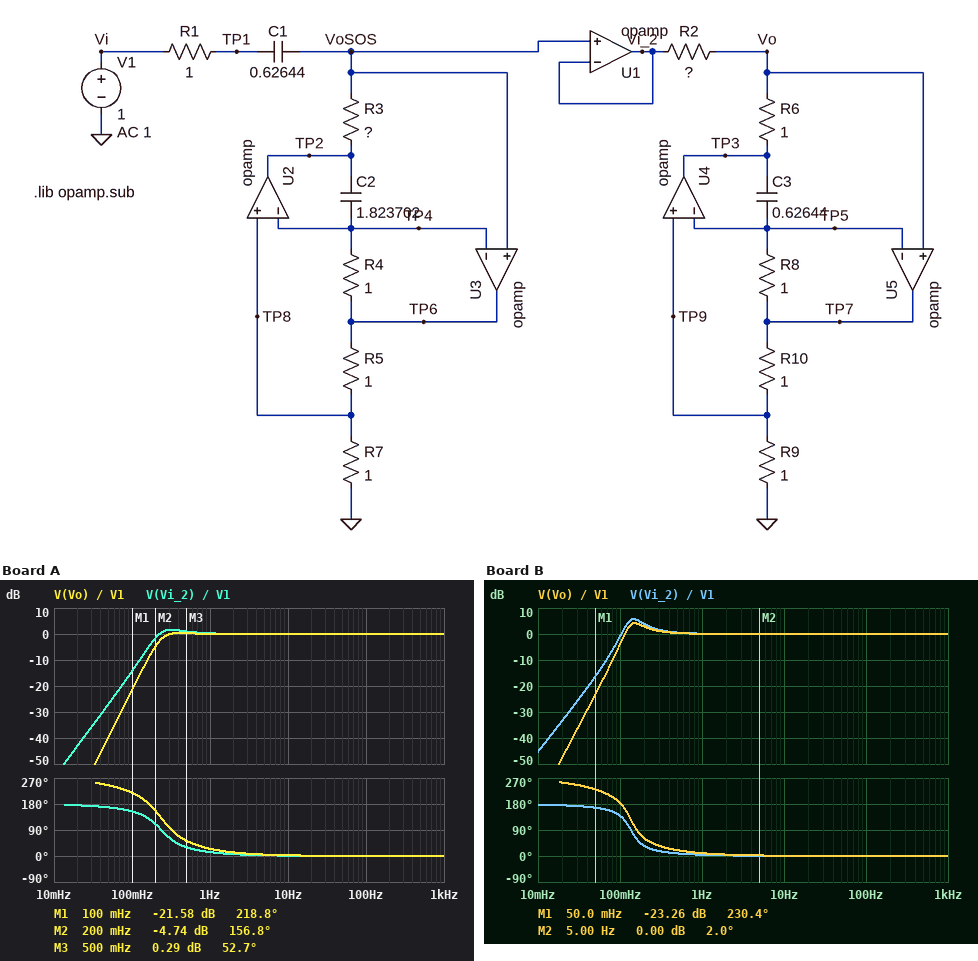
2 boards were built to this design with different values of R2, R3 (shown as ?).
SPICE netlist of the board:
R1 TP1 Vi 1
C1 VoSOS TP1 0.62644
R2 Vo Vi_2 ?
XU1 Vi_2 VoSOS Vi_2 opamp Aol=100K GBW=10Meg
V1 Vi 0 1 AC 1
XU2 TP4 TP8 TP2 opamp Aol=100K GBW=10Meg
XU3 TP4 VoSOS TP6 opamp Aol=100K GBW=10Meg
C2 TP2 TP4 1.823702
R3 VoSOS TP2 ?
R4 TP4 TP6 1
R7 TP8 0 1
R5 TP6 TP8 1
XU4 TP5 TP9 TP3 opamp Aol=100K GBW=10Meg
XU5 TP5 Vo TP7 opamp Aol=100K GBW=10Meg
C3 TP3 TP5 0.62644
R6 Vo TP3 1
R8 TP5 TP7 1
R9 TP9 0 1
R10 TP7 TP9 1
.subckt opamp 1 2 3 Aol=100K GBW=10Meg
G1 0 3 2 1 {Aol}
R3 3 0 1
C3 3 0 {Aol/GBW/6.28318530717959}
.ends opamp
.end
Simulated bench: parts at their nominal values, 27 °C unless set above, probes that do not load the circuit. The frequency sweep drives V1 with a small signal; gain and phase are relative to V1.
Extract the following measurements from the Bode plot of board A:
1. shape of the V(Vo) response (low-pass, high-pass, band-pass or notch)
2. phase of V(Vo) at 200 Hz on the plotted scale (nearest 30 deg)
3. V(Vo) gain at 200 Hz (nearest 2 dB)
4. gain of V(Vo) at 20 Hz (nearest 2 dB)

high-pass
0 deg
0 dB
0 dB
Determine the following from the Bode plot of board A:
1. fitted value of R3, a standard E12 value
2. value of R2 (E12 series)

0.39 Ω
0.82 Ω
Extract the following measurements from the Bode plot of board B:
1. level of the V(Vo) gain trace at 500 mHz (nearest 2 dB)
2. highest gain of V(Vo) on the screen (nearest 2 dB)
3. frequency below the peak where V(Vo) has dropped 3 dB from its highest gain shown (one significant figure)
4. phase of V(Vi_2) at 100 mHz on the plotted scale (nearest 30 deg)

0 dB
4 dB
100 mHz
150 deg
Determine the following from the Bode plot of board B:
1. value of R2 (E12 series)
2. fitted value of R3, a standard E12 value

0.39 Ω
1.2 Ω
